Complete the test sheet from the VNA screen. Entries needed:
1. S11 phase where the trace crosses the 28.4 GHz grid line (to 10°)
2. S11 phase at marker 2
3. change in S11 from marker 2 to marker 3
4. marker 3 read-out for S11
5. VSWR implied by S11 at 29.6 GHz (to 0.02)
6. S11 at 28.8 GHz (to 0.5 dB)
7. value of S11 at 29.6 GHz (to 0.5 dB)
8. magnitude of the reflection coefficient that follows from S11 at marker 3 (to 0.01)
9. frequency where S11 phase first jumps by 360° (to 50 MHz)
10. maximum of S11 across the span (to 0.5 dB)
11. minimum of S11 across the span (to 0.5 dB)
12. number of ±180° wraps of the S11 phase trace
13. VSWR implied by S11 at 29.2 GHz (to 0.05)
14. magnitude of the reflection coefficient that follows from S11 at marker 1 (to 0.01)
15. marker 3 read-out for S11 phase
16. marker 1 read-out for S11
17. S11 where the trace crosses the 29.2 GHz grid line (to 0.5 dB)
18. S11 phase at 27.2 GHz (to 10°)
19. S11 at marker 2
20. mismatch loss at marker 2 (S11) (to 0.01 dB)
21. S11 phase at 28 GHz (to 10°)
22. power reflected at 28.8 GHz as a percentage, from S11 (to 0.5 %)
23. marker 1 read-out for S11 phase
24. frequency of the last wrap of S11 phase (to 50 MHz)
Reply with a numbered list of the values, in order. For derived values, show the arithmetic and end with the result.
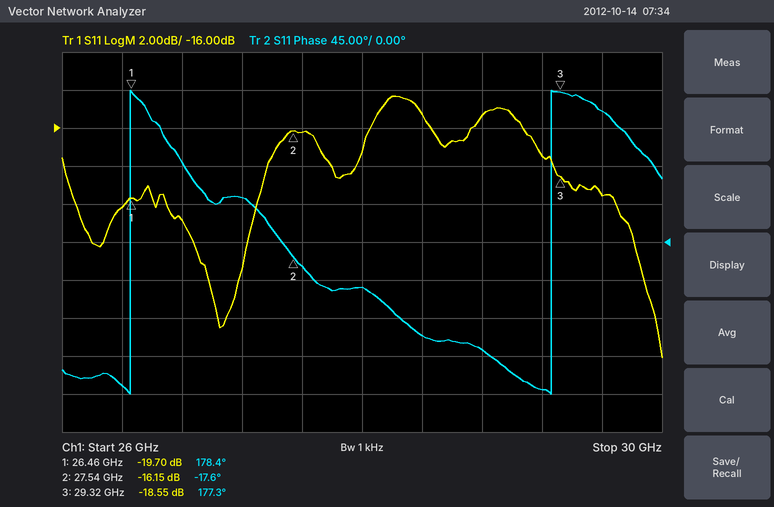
1. -110°
2. -17.6°
3. -18.55 − (-16.15) = -2.40 dB
4. -18.55 dB
5. |Γ| = 10^(-19.5/20) = 0.1059; VSWR = (1 + 0.1059)/(1 − 0.1059) ≈ 1.24
6. -15.5 dB
7. -19.5 dB
8. 10^(-18.55/20) ≈ 0.12
9. 26.45 GHz
10. -14.5 dB
11. -28.0 dB
12. 2
13. |Γ| = 10^(-17.5/20) = 0.1334; VSWR = (1 + 0.1334)/(1 − 0.1334) ≈ 1.31, so 1.30 to the nearest 0.05
14. 10^(-19.7/20) ≈ 0.10
15. 177.3°
16. -19.70 dB
17. -17.5 dB
18. 50°
19. -16.15 dB
20. −10 log10(1 − 10^(-16.15/10)) ≈ 0.11 dB
21. -50°
22. 10^(-15.5/10) ≈ 2.82 %, so 3.0 % to the nearest 0.5 %
23. 178.4°
24. 29.25 GHz
